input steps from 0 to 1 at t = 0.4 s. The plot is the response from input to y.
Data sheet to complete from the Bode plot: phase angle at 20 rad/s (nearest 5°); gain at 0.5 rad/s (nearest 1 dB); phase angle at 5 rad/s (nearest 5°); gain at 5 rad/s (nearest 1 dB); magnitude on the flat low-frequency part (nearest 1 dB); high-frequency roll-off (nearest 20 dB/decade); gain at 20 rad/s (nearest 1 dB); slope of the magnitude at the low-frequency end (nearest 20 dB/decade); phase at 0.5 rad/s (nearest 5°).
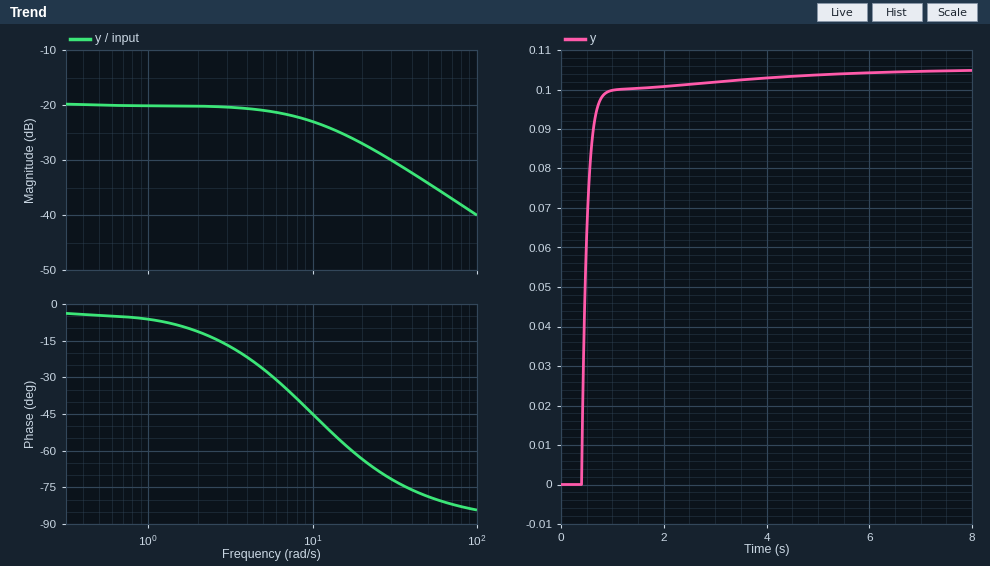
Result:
-65°
-20 dB
-25°
-21 dB
-20 dB
-20 dB/decade
-27 dB
0 dB/decade
-5°
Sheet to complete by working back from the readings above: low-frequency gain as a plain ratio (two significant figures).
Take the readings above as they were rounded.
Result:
0.10
